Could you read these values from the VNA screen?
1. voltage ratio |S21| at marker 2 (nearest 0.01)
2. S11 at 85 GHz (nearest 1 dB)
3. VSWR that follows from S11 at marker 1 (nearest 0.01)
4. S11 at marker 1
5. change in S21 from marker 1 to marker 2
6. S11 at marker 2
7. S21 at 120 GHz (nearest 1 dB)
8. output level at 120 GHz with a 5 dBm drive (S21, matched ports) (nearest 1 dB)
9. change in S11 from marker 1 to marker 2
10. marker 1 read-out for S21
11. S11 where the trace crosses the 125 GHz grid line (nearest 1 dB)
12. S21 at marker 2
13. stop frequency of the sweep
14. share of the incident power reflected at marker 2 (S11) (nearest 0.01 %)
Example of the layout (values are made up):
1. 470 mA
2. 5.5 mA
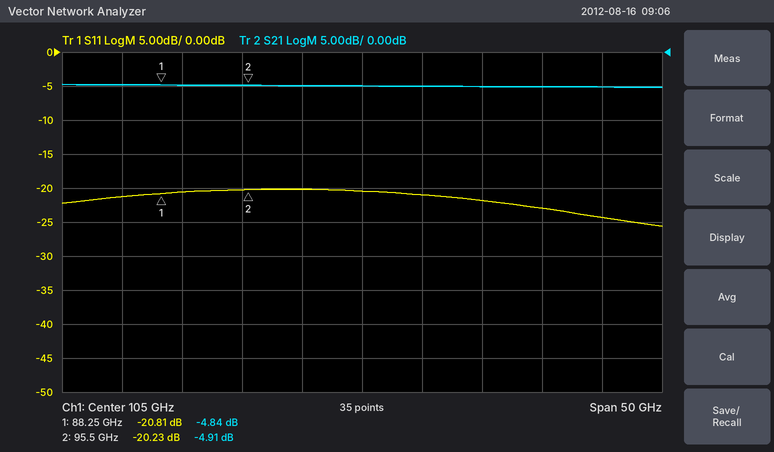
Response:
1. 0.57
2. -21 dB
3. 1.20
4. -20.81 dB
5. -0.07 dB
6. -20.23 dB
7. -5 dB
8. 0 dBm
9. 0.58 dB
10. -4.84 dB
11. -24 dB
12. -4.91 dB
13. 130 GHz
14. 0.95 %
